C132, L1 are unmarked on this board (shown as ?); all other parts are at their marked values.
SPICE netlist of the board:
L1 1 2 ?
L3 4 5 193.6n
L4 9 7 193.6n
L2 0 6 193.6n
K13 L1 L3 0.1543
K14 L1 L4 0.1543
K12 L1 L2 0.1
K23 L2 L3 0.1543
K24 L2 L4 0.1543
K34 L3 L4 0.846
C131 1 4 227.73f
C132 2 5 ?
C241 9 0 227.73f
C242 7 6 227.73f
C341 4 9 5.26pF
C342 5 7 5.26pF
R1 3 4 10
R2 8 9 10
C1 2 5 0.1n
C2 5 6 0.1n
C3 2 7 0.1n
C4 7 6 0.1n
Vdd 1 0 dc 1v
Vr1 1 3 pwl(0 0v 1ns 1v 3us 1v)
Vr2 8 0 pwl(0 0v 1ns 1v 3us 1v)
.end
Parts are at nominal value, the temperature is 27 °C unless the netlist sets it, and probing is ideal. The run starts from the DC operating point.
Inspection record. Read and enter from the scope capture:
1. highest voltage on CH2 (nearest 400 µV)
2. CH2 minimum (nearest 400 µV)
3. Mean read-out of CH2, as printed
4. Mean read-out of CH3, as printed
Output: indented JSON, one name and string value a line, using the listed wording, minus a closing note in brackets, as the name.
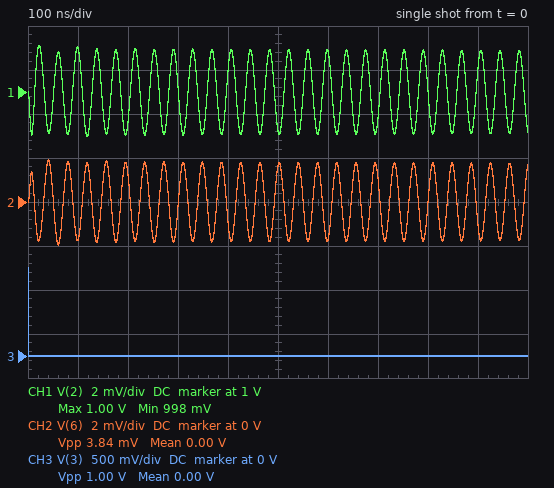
{
  "highest voltage on CH2": "2.0 mV",
  "CH2 minimum": "-2.0 mV",
  "Mean read-out of CH2, as printed": "0.00 V",
  "Mean read-out of CH3, as printed": "0.00 V"
}
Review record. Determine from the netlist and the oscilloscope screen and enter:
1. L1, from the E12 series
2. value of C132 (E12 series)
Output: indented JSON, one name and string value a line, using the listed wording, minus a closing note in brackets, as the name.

{
  "L1, from the E12 series": "220 nH",
  "value of C132": "470 fF"
}
